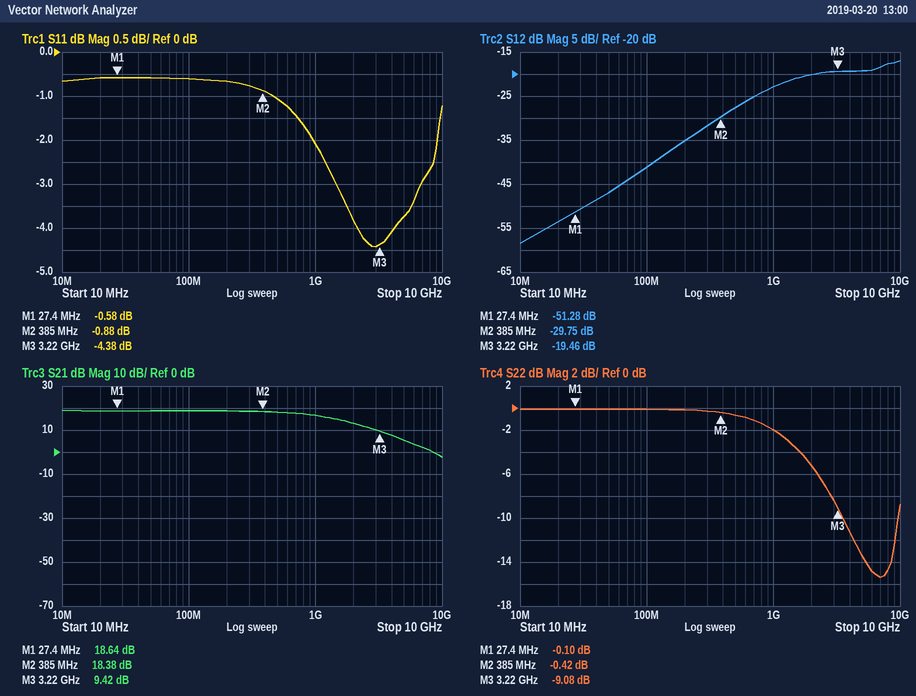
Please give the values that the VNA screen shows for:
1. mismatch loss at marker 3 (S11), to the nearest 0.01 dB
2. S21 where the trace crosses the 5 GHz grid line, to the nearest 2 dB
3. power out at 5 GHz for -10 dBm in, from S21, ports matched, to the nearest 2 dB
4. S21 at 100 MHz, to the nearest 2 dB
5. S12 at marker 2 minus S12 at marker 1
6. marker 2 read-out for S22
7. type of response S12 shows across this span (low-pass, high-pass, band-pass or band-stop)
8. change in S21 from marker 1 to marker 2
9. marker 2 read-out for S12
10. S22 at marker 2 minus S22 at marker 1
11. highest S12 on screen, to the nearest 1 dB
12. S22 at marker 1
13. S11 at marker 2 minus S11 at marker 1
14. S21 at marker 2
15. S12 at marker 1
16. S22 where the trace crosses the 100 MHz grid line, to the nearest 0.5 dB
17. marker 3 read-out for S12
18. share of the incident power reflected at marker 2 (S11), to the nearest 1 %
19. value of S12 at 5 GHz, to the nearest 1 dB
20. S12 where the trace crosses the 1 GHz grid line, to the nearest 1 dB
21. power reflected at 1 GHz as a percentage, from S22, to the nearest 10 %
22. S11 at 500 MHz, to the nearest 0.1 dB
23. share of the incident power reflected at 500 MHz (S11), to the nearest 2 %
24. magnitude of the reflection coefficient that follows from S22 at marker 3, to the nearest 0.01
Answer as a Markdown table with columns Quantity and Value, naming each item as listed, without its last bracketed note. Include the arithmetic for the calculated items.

| Quantity | Value |
|---|---|
| mismatch loss at marker 3 (S11), to the nearest 0.01 dB | −10 log10(1 − 10^(-4.38/10)) ≈ 1.97 dB |
| S21 where the trace crosses the 5 GHz grid line, to the nearest 2 dB | 6 dB |
| power out at 5 GHz for -10 dBm in, from S21, ports matched, to the nearest 2 dB | -10 dBm + (6 dB) = -4 dBm |
| S21 at 100 MHz, to the nearest 2 dB | 18 dB |
| S12 at marker 2 minus S12 at marker 1 | -29.75 − (-51.28) = 21.53 dB |
| marker 2 read-out for S22 | -0.42 dB |
| type of response S12 shows across this span | high-pass |
| change in S21 from marker 1 to marker 2 | 18.38 − (18.64) = -0.26 dB |
| marker 2 read-out for S12 | -29.75 dB |
| S22 at marker 2 minus S22 at marker 1 | -0.42 − (-0.1) = -0.32 dB |
| highest S12 on screen, to the nearest 1 dB | -17 dB |
| S22 at marker 1 | -0.10 dB |
| S11 at marker 2 minus S11 at marker 1 | -0.88 − (-0.58) = -0.30 dB |
| S21 at marker 2 | 18.38 dB |
| S12 at marker 1 | -51.28 dB |
| S22 where the trace crosses the 100 MHz grid line, to the nearest 0.5 dB | 0.0 dB |
| marker 3 read-out for S12 | -19.46 dB |
| share of the incident power reflected at marker 2 (S11), to the nearest 1 % | 10^(-0.88/10) ≈ 82 % |
| value of S12 at 5 GHz, to the nearest 1 dB | -19 dB |
| S12 where the trace crosses the 1 GHz grid line, to the nearest 1 dB | -23 dB |
| power reflected at 1 GHz as a percentage, from S22, to the nearest 10 % | 10^(-2/10) ≈ 63.1 %, so 60 % to the nearest 10 % |
| S11 at 500 MHz, to the nearest 0.1 dB | -1.1 dB |
| share of the incident power reflected at 500 MHz (S11), to the nearest 2 % | 10^(-1.1/10) ≈ 78 % |
| magnitude of the reflection coefficient that follows from S22 at marker 3, to the nearest 0.01 | 10^(-9.08/20) ≈ 0.35 |
